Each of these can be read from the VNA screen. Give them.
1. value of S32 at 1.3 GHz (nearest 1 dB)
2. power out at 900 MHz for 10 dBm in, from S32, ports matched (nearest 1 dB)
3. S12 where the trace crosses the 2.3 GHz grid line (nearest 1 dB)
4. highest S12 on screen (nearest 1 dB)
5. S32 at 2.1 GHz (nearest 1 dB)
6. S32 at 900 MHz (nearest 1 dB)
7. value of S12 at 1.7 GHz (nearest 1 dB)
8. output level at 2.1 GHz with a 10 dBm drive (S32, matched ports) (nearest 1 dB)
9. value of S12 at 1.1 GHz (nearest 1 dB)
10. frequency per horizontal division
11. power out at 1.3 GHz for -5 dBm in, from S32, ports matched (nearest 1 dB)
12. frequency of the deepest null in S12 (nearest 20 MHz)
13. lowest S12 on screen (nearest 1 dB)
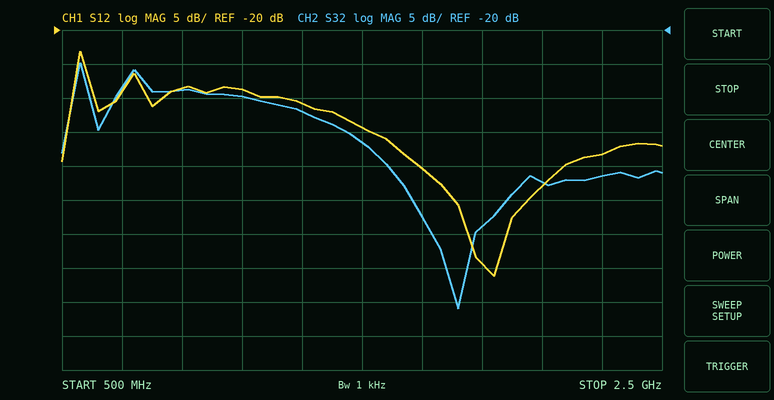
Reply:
-32 dB
-19 dBm
-38 dB
-23 dB
-42 dB
-29 dB
-40 dB
-32 dBm
-29 dB
200 MHz
-37 dBm
1.94 GHz
-56 dB
